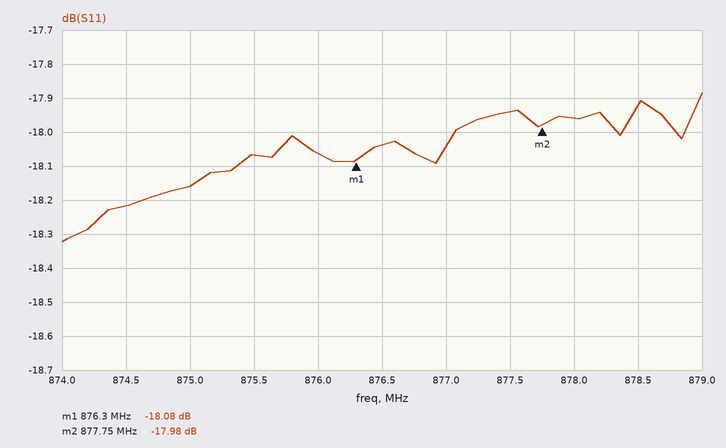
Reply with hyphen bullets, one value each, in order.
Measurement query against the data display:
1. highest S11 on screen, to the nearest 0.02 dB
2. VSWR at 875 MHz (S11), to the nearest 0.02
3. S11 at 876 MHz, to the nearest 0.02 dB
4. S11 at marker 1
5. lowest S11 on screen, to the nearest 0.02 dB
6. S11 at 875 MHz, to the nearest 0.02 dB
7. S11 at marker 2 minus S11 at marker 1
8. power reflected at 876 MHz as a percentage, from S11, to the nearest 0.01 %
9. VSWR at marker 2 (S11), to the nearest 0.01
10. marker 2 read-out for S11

- -17.88 dB
- 1.28
- -18.06 dB
- -18.08 dB
- -18.32 dB
- -18.16 dB
- 0.10 dB
- 1.56 %
- 1.29
- -17.98 dB
